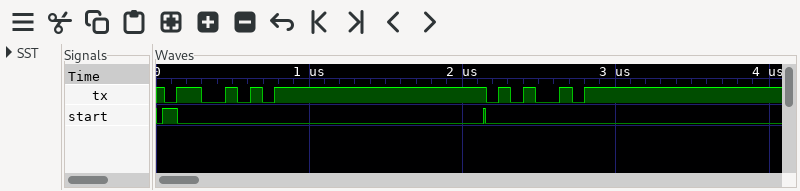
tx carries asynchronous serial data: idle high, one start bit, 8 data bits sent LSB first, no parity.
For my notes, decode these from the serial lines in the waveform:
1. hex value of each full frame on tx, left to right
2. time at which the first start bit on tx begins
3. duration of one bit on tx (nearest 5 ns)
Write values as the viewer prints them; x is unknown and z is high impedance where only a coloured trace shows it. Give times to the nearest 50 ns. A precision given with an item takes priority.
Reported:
53, A5
50 ns
80 ns
